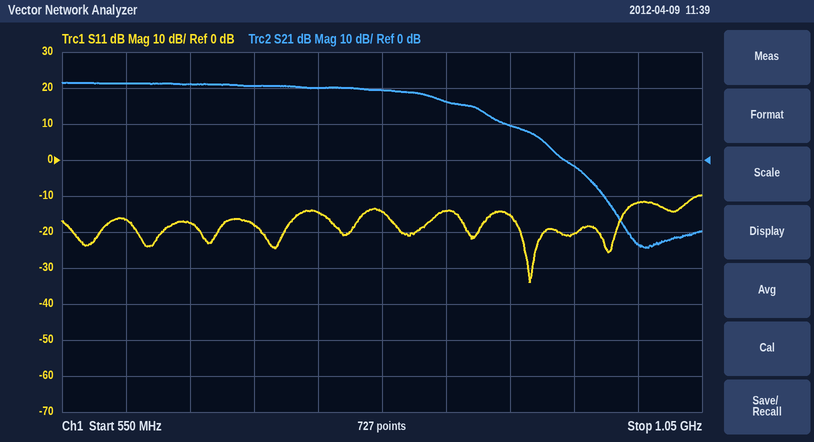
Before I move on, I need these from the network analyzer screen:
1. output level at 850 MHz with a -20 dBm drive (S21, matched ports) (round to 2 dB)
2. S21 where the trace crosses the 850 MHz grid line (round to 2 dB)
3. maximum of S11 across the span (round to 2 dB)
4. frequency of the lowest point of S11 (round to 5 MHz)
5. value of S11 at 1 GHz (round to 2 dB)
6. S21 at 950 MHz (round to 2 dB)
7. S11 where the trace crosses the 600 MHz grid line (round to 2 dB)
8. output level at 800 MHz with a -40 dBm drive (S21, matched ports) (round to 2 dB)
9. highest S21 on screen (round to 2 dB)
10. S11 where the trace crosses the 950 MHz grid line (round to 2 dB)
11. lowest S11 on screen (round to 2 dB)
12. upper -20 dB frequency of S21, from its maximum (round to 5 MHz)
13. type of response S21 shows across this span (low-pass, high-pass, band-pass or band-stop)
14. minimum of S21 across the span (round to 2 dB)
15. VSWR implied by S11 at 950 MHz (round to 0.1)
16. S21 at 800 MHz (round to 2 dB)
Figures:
-4 dBm
16 dB
-10 dB
915 MHz
-12 dB
-2 dB
-16 dB
-20 dBm
22 dB
-20 dB
-34 dB
935 MHz
low-pass
-24 dB
1.2
20 dB
